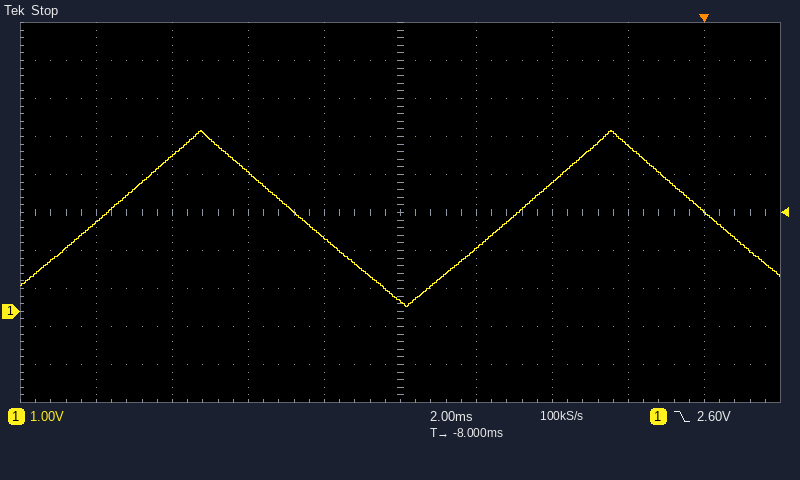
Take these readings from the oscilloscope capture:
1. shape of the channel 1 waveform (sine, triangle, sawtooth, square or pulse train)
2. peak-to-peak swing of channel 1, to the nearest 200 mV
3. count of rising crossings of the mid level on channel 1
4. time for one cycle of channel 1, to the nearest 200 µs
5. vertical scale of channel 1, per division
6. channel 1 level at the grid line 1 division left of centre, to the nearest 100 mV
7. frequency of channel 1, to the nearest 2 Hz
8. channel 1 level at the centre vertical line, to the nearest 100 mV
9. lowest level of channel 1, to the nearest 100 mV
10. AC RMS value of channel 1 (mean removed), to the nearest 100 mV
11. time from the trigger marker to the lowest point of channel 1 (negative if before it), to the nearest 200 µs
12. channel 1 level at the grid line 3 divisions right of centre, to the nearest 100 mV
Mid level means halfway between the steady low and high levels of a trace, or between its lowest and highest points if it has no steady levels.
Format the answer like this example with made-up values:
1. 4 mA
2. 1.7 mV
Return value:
1. triangle
2. 4.6 V
3. 2
4. 10.8 ms
5. 1 V
6. 1.9 V
7. 92 Hz
8. 300 mV
9. 100 mV
10. 1.3 V
11. -7.8 ms
12. 4.4 V
